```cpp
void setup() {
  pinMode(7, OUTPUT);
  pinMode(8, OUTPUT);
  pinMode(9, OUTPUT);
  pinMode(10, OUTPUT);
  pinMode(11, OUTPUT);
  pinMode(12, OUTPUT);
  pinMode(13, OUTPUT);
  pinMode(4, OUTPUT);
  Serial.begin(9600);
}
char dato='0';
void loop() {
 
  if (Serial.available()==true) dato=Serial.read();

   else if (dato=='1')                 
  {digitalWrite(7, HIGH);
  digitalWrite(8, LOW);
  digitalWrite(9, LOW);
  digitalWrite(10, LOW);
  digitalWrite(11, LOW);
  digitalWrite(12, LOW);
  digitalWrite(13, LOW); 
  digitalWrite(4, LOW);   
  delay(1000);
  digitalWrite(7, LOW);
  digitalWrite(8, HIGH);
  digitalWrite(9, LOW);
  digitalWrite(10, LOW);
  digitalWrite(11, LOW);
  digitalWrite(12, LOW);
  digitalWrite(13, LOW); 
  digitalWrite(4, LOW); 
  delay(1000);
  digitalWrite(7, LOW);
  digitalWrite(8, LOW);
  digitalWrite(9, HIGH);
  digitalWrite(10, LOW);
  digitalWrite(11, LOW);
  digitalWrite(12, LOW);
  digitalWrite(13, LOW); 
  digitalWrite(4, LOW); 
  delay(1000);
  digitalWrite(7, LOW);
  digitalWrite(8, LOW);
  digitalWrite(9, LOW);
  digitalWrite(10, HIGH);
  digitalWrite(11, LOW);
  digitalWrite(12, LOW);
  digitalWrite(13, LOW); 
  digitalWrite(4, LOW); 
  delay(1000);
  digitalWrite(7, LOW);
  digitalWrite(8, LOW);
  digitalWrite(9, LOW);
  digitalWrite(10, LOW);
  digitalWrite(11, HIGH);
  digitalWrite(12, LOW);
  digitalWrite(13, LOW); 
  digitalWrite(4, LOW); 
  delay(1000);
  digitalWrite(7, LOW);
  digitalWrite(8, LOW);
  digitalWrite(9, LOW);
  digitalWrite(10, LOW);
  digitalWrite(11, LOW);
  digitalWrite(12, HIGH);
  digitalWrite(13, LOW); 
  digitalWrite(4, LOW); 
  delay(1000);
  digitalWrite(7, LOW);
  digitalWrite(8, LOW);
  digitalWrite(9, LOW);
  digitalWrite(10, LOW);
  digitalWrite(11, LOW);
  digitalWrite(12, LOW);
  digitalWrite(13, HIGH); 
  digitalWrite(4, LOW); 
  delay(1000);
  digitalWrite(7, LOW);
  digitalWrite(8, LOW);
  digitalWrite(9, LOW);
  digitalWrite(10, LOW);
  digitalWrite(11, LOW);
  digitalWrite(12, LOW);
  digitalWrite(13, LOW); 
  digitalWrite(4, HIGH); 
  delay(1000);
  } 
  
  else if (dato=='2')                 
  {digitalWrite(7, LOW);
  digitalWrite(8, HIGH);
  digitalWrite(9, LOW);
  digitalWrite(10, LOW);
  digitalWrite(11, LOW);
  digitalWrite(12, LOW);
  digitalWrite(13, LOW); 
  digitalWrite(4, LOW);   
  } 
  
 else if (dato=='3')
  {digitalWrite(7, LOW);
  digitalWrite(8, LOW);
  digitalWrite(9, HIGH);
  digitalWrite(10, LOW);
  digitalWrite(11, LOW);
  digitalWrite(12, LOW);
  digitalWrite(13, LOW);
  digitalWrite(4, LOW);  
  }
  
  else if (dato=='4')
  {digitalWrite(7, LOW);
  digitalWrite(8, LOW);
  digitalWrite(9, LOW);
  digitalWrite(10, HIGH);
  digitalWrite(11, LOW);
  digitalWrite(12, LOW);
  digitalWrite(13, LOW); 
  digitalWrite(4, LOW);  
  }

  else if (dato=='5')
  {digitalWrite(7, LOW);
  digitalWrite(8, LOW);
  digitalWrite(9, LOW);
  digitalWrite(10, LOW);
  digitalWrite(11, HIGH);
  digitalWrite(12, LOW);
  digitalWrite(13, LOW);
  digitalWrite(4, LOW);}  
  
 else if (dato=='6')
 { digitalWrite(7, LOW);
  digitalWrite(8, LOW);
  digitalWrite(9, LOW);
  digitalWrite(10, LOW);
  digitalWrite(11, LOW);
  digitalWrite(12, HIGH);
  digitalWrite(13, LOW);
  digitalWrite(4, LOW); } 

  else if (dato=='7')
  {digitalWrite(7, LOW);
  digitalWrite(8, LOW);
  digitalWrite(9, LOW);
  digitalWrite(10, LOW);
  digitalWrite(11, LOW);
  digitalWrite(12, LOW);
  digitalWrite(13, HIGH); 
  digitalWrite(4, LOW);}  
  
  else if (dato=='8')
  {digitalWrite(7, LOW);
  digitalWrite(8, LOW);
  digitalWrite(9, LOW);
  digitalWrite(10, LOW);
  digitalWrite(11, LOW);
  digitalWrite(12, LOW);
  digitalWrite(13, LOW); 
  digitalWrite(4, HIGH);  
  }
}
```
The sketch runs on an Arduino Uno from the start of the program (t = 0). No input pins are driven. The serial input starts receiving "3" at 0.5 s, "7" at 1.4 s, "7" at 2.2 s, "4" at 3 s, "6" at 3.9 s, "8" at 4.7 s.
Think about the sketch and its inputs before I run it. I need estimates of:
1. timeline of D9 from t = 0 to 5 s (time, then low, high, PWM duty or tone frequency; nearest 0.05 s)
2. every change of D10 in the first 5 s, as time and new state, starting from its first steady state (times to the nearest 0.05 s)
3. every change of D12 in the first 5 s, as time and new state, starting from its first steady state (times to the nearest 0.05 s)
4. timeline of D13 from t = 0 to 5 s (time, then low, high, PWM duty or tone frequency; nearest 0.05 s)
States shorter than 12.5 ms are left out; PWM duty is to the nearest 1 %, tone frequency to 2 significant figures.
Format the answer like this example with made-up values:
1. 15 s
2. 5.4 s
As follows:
1. 0 s low; 0.5 s high; 1.4 s low
2. 0 s low; 3 s high; 3.9 s low
3. 0 s low; 3.9 s high; 4.7 s low
4. 0 s low; 1.4 s high; 3 s low
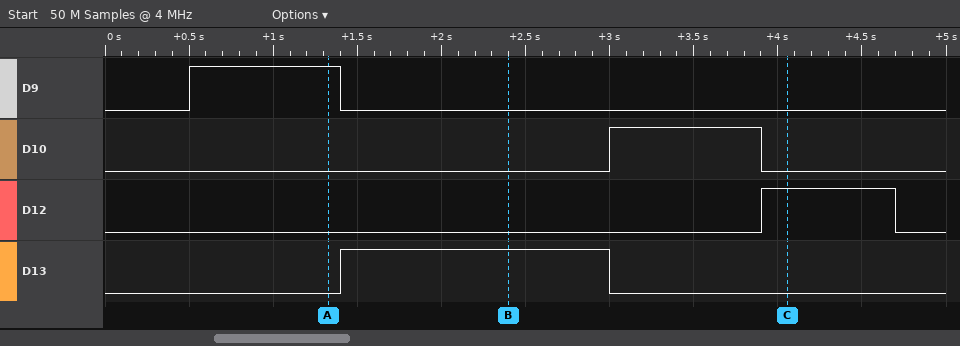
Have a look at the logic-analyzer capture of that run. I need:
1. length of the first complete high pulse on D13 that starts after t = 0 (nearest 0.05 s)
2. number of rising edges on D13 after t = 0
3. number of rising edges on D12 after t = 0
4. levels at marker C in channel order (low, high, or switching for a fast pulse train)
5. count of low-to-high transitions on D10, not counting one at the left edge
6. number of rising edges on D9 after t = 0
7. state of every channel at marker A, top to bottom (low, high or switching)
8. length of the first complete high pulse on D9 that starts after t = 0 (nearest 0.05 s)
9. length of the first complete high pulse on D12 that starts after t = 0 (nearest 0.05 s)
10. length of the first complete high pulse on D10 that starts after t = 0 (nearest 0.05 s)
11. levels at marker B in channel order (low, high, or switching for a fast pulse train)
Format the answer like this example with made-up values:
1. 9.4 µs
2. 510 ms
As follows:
1. 1.60 s
2. 1
3. 1
4. D9 low, D10 low, D12 high, D13 low
5. 1
6. 1
7. D9 high, D10 low, D12 low, D13 low
8. 0.90 s
9. 0.80 s
10. 0.90 s
11. D9 low, D10 low, D12 low, D13 high
